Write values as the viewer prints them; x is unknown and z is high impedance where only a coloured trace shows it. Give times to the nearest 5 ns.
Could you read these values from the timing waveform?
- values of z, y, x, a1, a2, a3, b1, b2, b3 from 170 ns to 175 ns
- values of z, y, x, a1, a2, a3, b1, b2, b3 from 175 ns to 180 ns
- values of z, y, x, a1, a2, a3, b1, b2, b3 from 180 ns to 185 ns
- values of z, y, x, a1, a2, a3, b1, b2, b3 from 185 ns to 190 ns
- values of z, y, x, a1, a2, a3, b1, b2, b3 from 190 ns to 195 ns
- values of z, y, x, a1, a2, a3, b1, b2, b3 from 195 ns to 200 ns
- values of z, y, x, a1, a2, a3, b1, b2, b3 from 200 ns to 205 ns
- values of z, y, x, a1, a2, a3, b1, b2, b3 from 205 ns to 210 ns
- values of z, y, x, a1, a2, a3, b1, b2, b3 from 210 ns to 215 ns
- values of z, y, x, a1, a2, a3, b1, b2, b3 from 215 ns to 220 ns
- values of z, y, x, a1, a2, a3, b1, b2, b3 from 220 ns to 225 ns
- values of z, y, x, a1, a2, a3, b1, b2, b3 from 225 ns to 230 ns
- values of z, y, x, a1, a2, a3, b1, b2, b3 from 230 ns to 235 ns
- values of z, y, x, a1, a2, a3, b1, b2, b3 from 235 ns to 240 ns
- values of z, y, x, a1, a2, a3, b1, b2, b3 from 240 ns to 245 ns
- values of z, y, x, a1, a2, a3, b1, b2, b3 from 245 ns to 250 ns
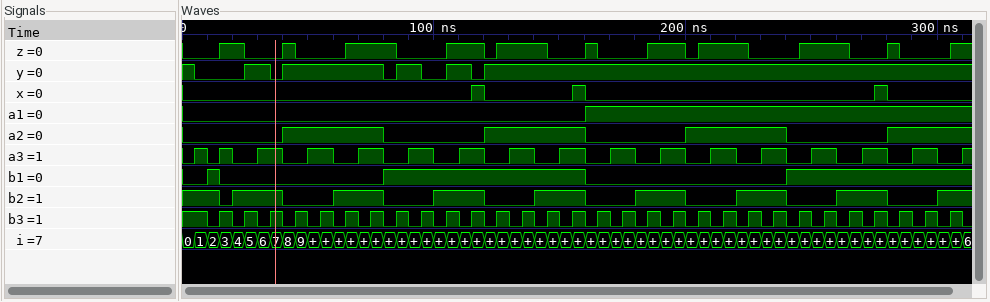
z=0, y=1, x=0, a1=1, a2=0, a3=1, b1=0, b2=0, b3=0
z=0, y=1, x=0, a1=1, a2=0, a3=1, b1=0, b2=0, b3=1
z=0, y=1, x=0, a1=1, a2=0, a3=0, b1=0, b2=1, b3=0
z=1, y=1, x=0, a1=1, a2=0, a3=0, b1=0, b2=1, b3=1
z=1, y=1, x=0, a1=1, a2=0, a3=1, b1=0, b2=1, b3=0
z=1, y=1, x=0, a1=1, a2=0, a3=1, b1=0, b2=1, b3=1
z=0, y=1, x=0, a1=1, a2=1, a3=0, b1=0, b2=0, b3=0
z=1, y=1, x=0, a1=1, a2=1, a3=0, b1=0, b2=0, b3=1
z=1, y=1, x=0, a1=1, a2=1, a3=1, b1=0, b2=0, b3=0
z=1, y=1, x=0, a1=1, a2=1, a3=1, b1=0, b2=0, b3=1
z=1, y=1, x=0, a1=1, a2=1, a3=0, b1=0, b2=1, b3=0
z=0, y=1, x=0, a1=1, a2=1, a3=0, b1=0, b2=1, b3=1
z=0, y=1, x=0, a1=1, a2=1, a3=1, b1=0, b2=1, b3=0
z=0, y=1, x=0, a1=1, a2=1, a3=1, b1=0, b2=1, b3=1
z=0, y=1, x=0, a1=1, a2=0, a3=0, b1=1, b2=0, b3=0
z=1, y=1, x=0, a1=1, a2=0, a3=0, b1=1, b2=0, b3=1
